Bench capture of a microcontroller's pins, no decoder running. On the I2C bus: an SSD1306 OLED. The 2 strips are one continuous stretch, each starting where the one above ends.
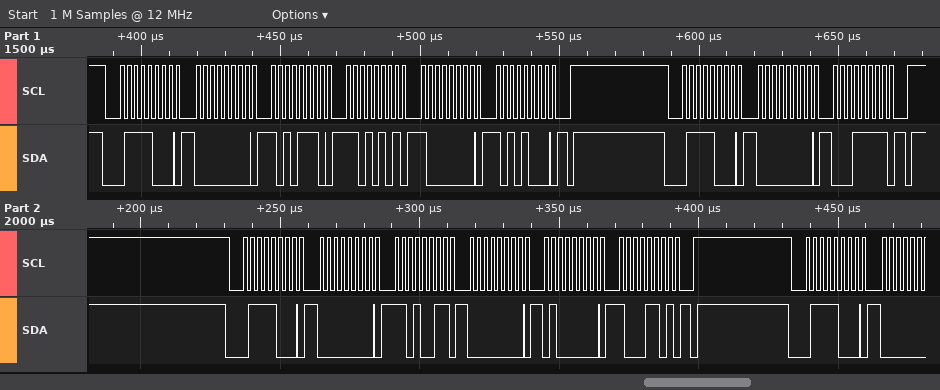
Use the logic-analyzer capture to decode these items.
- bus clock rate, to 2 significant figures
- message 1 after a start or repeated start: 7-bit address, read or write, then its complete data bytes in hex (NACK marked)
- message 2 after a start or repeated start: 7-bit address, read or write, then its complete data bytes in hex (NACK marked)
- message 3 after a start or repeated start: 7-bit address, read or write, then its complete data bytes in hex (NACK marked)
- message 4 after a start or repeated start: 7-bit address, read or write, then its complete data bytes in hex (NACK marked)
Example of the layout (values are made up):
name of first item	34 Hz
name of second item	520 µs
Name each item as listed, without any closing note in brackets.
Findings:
bus clock rate, to 2 significant figures	400 kHz
message 1 after a start or repeated start: 7-bit address, read or write, then its complete data bytes in hex	0x3C write: 00 AE D5 80 A8
message 2 after a start or repeated start: 7-bit address, read or write, then its complete data bytes in hex	0x3C write: 00 1F
message 3 after a start or repeated start: 7-bit address, read or write, then its complete data bytes in hex	0x3C write: 00 D3 00 40 8D
message 4 after a start or repeated start: 7-bit address, read or write, then its complete data bytes in hex	0x3C write
